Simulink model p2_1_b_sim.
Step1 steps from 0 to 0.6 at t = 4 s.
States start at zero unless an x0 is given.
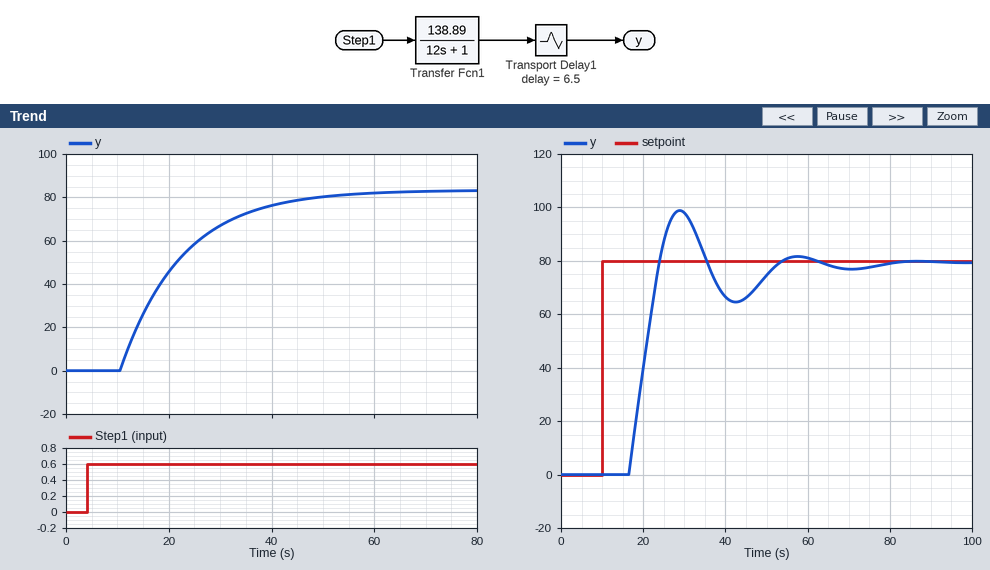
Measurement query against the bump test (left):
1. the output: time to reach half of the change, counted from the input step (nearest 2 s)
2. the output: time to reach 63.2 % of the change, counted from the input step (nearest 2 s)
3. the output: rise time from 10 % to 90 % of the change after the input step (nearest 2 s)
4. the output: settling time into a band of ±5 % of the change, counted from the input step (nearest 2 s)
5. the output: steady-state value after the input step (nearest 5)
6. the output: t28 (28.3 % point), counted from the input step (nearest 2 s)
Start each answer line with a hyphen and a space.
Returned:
- 14 s
- 18 s
- 26 s
- 42 s
- 85
- 10 s
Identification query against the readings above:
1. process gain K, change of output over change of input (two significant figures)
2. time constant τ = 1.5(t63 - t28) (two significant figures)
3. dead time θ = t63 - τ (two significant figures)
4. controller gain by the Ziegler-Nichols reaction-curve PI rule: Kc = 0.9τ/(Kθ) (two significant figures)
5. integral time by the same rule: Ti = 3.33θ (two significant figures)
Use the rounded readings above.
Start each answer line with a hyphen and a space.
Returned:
- 140
- 12 s
- 6.0 s
- 0.013
- 20 s
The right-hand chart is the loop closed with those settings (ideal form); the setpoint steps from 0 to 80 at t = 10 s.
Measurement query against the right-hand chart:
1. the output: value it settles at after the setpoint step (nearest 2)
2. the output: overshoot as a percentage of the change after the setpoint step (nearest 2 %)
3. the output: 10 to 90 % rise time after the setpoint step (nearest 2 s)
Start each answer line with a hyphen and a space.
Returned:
- 80
- 24 %
- 6 s
